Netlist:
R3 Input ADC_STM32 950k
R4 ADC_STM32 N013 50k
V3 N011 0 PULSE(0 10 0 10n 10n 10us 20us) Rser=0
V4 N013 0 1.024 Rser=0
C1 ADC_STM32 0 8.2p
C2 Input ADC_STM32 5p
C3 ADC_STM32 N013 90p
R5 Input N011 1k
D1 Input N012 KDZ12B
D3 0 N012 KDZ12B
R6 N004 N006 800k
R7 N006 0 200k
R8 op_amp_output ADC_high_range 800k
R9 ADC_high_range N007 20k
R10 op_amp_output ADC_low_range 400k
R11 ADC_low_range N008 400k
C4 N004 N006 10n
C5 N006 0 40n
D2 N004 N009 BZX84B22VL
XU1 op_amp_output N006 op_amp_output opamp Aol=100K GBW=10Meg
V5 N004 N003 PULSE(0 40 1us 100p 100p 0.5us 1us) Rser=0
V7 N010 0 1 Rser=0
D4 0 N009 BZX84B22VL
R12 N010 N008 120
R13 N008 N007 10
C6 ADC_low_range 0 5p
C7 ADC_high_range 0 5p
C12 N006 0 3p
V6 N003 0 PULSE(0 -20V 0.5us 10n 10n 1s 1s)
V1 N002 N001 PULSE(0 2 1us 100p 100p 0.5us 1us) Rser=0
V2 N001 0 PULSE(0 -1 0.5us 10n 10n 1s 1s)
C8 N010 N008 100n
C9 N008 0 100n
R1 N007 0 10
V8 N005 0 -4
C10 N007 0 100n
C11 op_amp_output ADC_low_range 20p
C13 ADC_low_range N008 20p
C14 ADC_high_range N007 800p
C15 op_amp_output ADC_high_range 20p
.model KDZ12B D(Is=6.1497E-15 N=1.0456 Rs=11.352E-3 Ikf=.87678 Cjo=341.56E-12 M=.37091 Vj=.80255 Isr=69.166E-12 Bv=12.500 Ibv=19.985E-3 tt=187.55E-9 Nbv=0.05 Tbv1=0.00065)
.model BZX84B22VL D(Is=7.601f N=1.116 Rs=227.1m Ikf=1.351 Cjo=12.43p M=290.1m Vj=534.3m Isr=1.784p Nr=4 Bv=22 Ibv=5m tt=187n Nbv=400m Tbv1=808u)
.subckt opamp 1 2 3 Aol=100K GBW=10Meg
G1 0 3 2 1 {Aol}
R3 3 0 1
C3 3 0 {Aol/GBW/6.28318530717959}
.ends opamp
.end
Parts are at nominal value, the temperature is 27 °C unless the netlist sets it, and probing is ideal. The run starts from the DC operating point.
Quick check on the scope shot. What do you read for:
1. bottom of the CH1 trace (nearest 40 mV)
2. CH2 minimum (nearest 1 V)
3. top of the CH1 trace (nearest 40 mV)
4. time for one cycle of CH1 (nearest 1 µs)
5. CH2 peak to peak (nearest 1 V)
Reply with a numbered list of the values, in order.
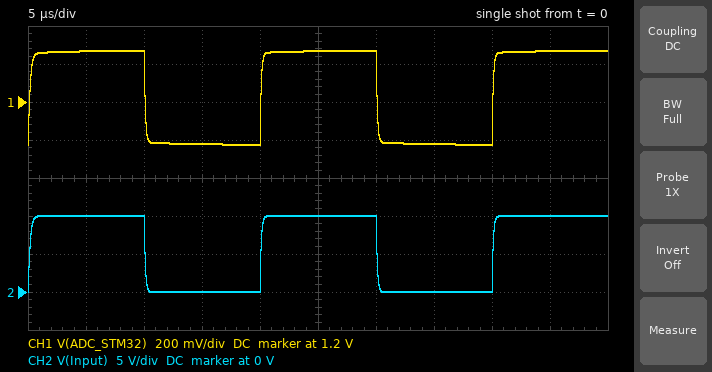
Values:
1. 960 mV
2. 0 V
3. 1.48 V
4. 20 µs
5. 10 V
